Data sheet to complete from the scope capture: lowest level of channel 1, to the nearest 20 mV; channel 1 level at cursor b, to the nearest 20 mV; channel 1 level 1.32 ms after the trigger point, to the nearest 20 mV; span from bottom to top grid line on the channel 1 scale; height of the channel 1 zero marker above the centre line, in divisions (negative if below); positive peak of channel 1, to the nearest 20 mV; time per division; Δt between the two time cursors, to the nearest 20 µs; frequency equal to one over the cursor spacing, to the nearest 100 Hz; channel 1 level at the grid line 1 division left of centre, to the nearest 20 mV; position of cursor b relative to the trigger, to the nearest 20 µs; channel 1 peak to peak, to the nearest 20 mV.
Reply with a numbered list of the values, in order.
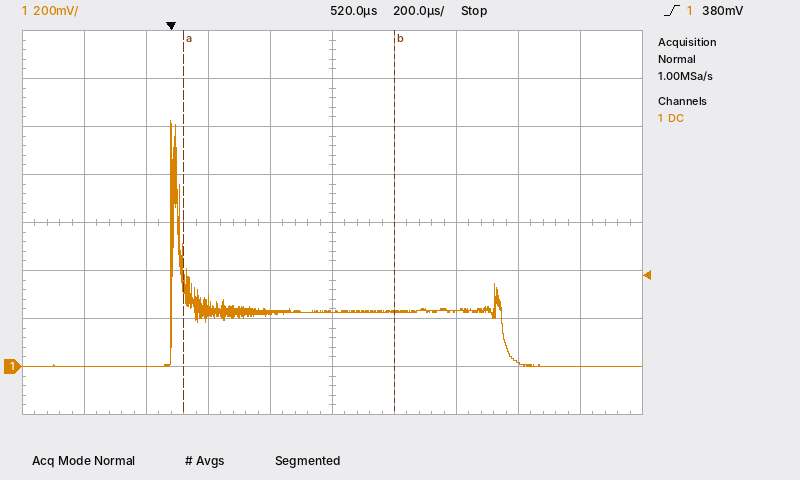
1. 0 mV
2. 220 mV
3. 0 mV
4. 1.6 V
5. -3.0 div
6. 1.02 V
7. 200 µs
8. 680 µs
9. 1.5 kHz
10. 220 mV
11. +720 µs
12. 1.02 V
